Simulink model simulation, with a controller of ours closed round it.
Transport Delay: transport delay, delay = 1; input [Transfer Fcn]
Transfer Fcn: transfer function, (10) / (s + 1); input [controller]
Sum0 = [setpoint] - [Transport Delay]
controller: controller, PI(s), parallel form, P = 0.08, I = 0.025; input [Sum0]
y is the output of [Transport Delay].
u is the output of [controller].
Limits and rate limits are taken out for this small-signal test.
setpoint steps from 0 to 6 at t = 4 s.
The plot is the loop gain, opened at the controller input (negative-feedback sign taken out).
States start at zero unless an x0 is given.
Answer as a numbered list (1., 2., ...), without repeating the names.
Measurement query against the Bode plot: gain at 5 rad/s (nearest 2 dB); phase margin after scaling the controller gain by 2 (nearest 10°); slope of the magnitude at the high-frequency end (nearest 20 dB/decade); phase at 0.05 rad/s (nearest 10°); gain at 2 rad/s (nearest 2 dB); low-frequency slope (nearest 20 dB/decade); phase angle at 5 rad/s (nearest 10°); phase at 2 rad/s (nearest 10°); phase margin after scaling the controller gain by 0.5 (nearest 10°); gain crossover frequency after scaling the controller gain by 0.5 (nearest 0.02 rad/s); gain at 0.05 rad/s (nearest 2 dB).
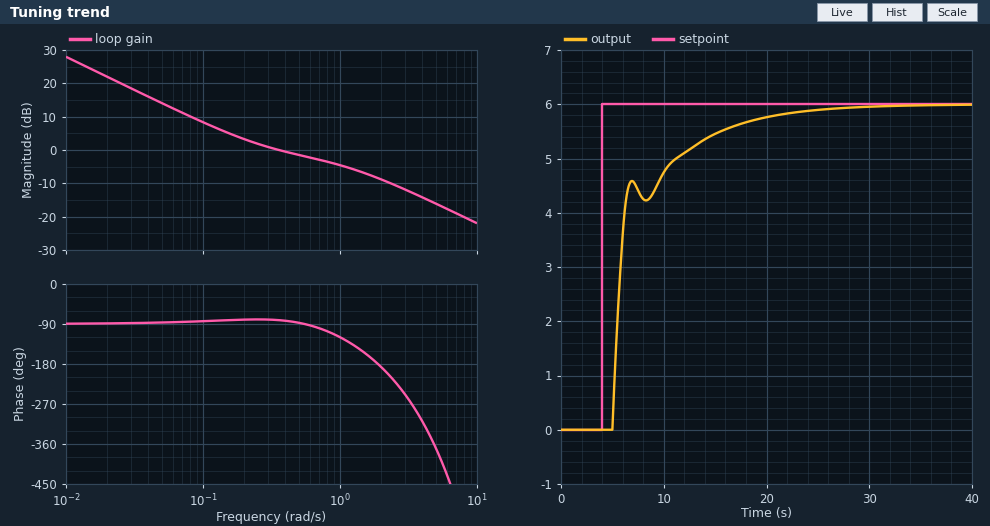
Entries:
1. -16 dB
2. 40°
3. -20 dB/decade
4. -90°
5. -8 dB
6. -20 dB/decade
7. -370°
8. -190°
9. 100°
10. 0.14 rad/s
11. 14 dB
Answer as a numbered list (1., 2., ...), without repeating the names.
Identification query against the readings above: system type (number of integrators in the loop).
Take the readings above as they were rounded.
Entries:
1. 1
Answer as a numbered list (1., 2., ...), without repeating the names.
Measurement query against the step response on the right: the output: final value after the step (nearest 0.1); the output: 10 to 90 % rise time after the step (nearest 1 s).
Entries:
1. 6.0
2. 9 s
